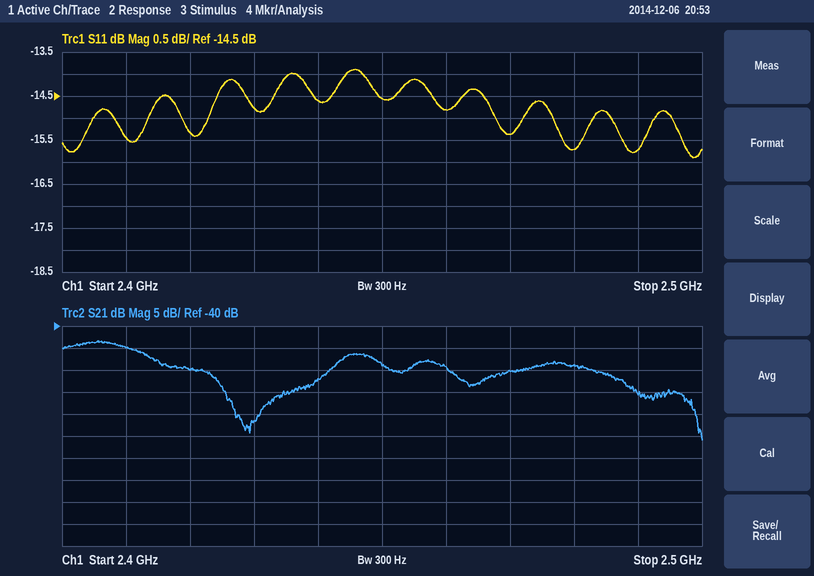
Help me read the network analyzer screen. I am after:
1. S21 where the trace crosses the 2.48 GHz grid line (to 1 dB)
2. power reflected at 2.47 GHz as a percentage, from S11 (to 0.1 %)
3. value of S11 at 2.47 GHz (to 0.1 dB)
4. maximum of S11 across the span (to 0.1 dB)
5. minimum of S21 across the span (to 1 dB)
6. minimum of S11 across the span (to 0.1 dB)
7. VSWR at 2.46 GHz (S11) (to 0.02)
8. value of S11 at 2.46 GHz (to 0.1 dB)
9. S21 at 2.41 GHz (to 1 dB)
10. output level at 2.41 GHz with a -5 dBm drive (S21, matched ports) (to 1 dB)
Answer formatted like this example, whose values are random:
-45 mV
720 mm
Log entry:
-49 dB
2.9 %
-15.4 dB
-13.9 dB
-66 dB
-15.9 dB
1.44
-14.8 dB
-45 dB
-50 dBm
